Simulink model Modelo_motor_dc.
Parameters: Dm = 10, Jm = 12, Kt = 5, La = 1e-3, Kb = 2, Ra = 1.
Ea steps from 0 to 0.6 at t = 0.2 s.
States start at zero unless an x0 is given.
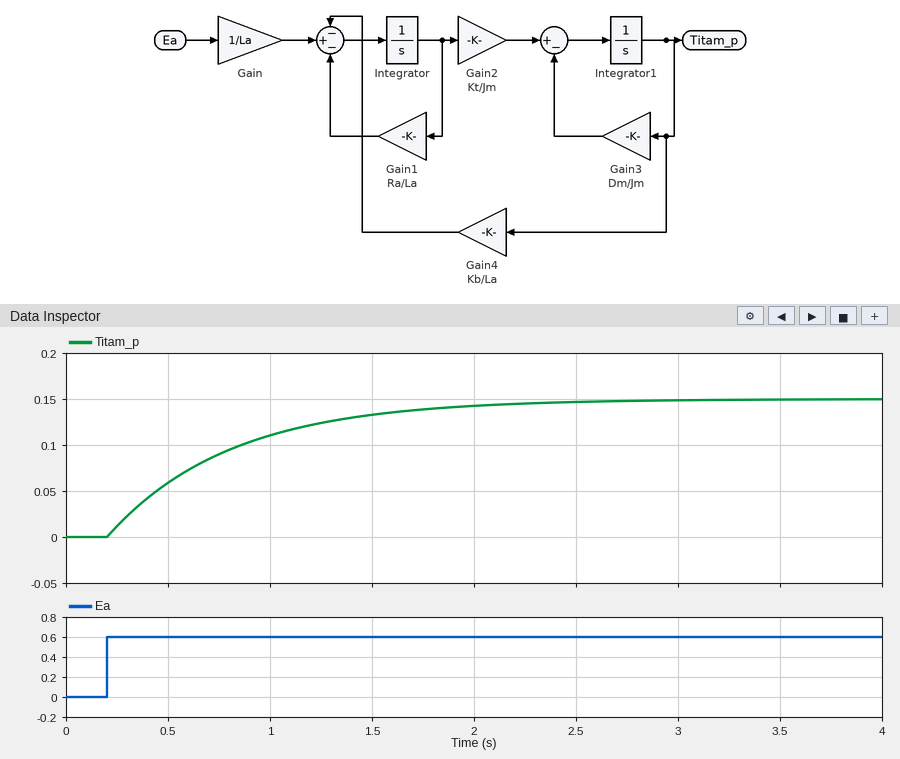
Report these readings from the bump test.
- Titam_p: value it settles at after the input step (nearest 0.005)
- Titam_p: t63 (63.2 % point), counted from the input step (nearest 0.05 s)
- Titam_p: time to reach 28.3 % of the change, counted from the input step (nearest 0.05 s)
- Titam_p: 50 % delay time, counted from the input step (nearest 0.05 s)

0.150
0.60 s
0.20 s
0.40 s
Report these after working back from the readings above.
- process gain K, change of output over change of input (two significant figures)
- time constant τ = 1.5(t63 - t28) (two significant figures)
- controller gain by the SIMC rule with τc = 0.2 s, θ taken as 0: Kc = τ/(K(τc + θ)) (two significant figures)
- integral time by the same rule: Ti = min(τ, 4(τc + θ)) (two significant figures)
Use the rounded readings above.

0.25
0.60 s
12
0.60 s
